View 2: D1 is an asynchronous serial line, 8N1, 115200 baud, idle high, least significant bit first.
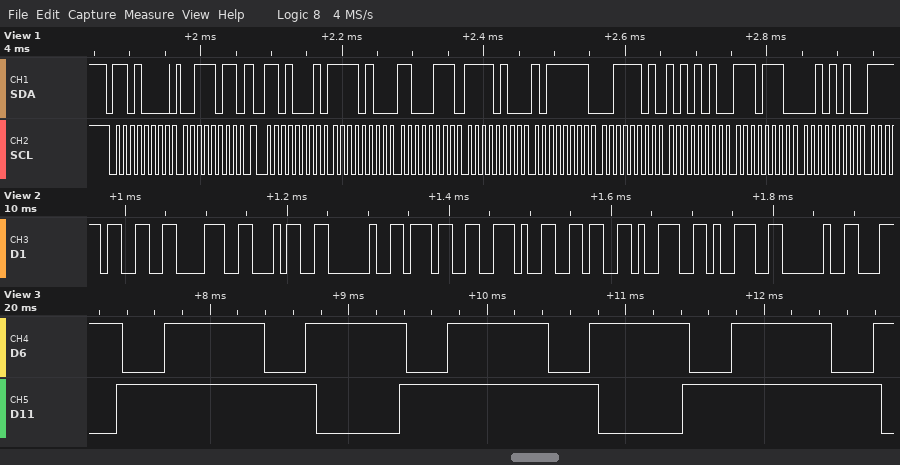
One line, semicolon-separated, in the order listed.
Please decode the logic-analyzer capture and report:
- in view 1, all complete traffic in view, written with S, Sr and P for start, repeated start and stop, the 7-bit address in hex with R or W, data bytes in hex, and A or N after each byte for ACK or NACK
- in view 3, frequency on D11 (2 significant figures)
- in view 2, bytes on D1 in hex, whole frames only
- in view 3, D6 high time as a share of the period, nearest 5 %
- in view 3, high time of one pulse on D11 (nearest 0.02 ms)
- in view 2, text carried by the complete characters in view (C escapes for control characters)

S 68W A 3B A Sr 68R A F4 A C7 A F4 A BF A 3D A AA A EE A 2A A; 490 Hz; 0x33 0x38 0x34 0x20 0x37 0x2E 0x36 0x39 0x39 0x20; 70 %; 1.44 ms; "384 7.699 "
